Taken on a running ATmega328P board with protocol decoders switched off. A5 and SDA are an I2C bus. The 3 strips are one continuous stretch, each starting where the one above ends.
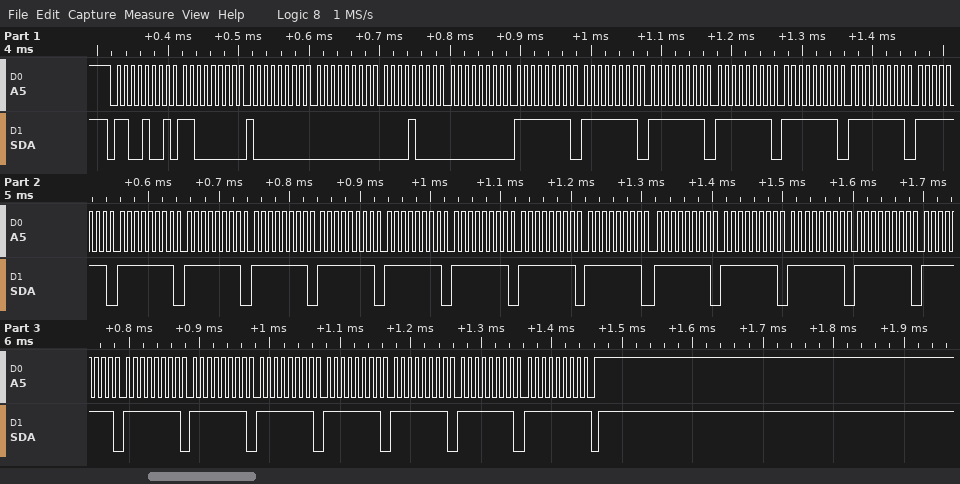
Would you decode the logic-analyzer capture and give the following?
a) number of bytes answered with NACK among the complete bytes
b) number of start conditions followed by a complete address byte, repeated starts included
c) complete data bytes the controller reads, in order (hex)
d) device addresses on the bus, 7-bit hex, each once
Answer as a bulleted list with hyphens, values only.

- 1
- 1
- C0 80 00 08 00 FF FF FF FF FF FF FF FF FF FF FF FF FF FF FF FF FF FF FF FF FF FF FF FF FF FF FF
- 0x64
